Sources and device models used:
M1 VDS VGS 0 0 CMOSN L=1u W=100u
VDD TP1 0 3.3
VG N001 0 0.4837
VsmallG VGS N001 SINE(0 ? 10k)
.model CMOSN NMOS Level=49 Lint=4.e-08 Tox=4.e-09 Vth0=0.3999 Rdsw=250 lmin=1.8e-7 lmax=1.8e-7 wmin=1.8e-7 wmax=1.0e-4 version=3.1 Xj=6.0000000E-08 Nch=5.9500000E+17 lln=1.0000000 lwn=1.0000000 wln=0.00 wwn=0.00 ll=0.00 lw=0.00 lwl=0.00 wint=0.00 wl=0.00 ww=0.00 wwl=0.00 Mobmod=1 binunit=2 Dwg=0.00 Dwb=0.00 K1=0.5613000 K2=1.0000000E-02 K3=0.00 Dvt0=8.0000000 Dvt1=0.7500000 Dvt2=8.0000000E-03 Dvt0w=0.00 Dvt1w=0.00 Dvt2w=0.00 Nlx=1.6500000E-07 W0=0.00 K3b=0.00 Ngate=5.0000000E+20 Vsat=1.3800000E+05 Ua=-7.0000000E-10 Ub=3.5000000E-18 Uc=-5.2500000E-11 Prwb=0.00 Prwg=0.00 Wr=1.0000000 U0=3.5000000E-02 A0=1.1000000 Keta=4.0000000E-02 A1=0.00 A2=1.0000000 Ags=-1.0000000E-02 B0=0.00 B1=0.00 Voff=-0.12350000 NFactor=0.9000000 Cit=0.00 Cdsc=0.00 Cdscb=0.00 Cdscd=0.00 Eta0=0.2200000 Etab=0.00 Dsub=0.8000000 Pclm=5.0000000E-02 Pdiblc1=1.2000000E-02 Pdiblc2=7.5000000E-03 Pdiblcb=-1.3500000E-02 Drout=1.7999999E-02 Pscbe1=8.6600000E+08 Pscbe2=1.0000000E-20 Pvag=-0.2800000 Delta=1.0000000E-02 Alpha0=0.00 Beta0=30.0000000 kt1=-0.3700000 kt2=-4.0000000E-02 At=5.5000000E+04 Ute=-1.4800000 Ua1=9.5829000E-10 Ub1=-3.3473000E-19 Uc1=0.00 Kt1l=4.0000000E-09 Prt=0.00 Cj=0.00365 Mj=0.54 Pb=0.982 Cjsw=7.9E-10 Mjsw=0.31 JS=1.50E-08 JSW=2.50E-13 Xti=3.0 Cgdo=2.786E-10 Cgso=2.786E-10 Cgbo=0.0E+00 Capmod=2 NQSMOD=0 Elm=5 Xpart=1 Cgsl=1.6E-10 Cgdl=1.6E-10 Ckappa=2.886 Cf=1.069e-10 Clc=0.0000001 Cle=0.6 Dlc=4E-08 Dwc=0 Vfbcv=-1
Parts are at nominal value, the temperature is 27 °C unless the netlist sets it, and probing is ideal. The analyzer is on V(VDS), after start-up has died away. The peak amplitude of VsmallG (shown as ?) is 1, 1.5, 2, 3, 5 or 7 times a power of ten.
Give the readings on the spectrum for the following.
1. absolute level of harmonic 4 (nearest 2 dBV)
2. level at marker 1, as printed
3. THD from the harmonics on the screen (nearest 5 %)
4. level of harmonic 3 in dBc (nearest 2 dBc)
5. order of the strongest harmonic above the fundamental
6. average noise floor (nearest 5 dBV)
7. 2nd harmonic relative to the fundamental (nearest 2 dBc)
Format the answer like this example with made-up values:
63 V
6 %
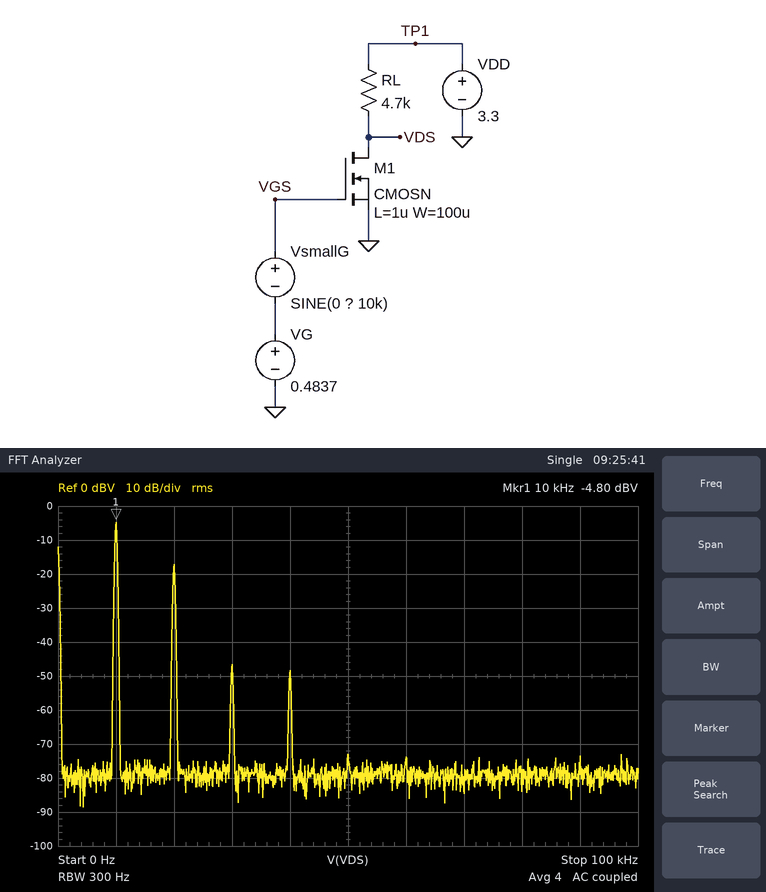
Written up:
-48 dBV
-4.80 dBV
25 %
-42 dBc
2
-80 dBV
-12 dBc
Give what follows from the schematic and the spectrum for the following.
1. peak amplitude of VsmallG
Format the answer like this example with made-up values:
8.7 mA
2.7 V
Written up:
100 mV
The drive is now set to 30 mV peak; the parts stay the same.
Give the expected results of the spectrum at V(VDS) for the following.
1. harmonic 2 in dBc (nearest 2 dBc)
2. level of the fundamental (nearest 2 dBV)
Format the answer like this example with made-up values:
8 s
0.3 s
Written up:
-22 dBc
-16 dBV
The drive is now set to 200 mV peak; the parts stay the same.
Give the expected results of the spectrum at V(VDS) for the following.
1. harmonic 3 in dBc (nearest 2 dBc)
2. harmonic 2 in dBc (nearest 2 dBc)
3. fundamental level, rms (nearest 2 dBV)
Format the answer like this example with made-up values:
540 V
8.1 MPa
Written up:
-38 dBc
-10 dBc
2 dBV
